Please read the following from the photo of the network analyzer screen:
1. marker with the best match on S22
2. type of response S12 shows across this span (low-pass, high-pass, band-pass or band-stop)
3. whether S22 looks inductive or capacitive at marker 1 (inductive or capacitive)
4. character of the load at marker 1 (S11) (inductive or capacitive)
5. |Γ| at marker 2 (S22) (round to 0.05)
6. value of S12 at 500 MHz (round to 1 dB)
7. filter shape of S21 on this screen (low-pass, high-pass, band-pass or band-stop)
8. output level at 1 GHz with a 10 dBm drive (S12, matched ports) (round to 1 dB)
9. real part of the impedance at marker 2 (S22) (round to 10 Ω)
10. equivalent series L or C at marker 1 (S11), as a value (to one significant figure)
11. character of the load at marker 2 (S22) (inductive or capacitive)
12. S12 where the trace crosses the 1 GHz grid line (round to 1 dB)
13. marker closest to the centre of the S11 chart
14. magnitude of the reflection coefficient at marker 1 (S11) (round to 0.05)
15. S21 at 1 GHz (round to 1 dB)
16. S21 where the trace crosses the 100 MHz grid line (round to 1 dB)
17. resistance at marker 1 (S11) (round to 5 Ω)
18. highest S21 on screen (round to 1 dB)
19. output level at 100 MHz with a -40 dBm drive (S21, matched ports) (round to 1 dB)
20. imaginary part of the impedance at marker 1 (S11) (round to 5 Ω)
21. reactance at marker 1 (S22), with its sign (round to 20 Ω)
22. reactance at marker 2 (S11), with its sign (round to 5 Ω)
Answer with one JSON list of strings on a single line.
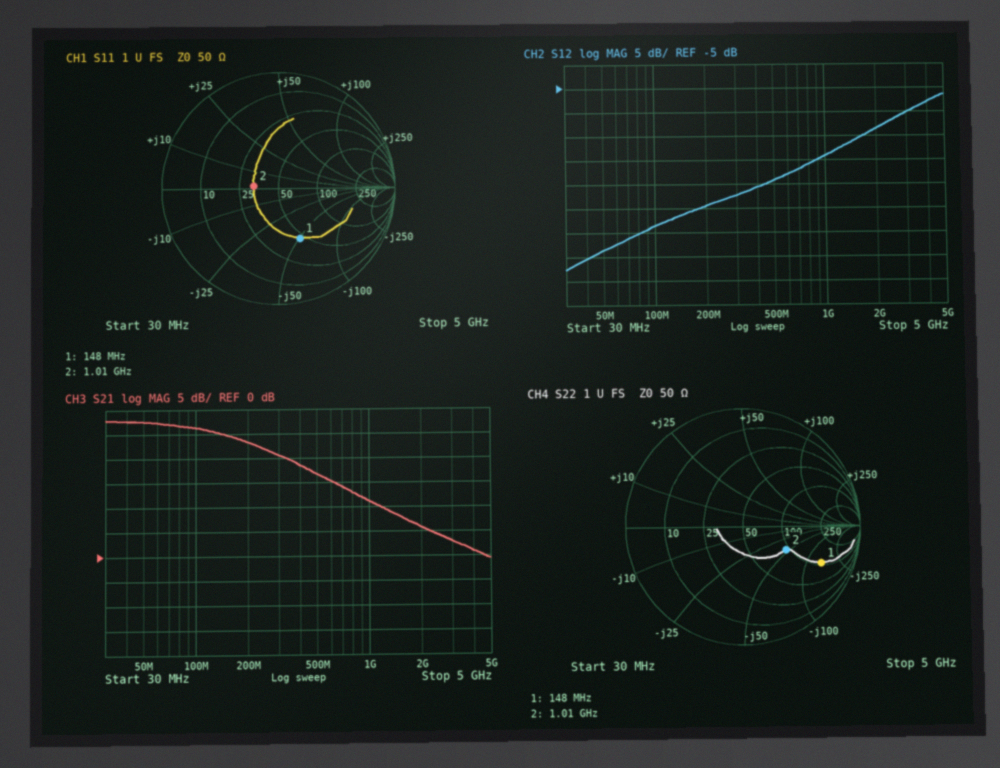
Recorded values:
["marker 2", "high-pass", "capacitive", "capacitive", "0.40", "-24 dB", "low-pass", "-9 dBm", "90 Ω", "20 pF", "capacitive", "-19 dB", "marker 2", "0.45", "11 dB", "26 dB", "45 Ω", "28 dB", "-14 dBm", "-50 Ω", "-140 Ω", "0 Ω"]
